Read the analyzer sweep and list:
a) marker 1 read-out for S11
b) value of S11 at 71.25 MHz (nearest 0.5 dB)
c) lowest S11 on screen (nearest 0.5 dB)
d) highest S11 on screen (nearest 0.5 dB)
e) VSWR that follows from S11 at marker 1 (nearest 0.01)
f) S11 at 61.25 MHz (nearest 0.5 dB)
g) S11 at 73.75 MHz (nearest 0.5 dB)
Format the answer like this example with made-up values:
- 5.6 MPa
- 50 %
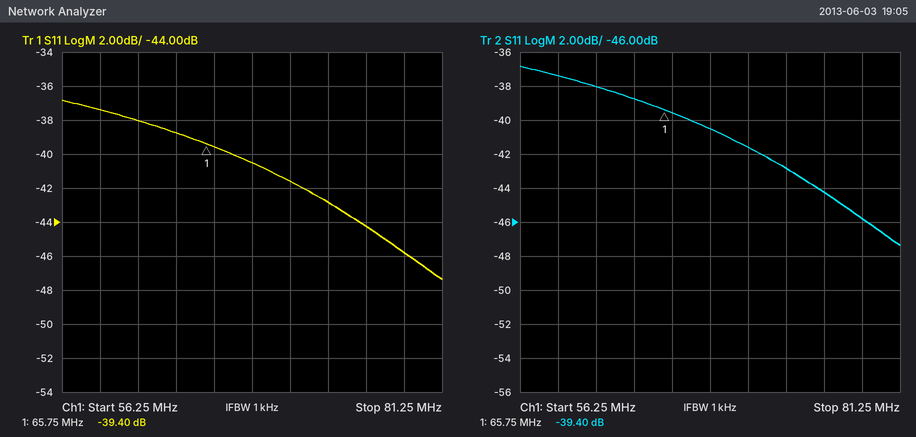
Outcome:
- -39.40 dB
- -41.5 dB
- -47.5 dB
- -37.0 dB
- 1.02
- -38.0 dB
- -43.0 dB
